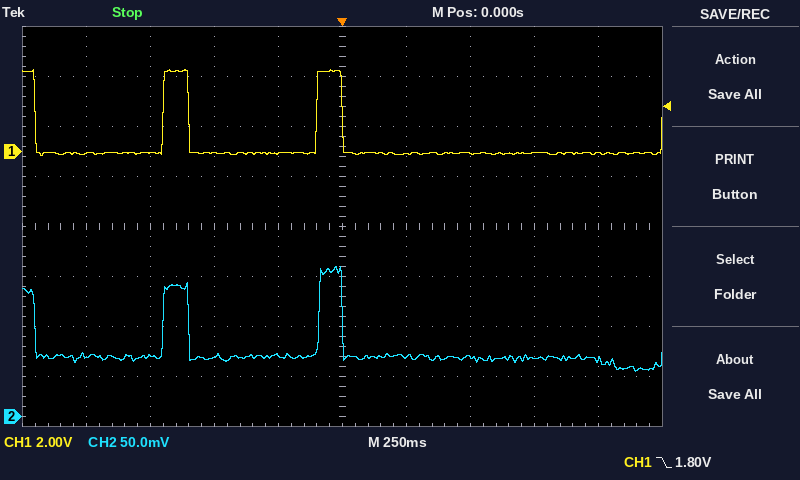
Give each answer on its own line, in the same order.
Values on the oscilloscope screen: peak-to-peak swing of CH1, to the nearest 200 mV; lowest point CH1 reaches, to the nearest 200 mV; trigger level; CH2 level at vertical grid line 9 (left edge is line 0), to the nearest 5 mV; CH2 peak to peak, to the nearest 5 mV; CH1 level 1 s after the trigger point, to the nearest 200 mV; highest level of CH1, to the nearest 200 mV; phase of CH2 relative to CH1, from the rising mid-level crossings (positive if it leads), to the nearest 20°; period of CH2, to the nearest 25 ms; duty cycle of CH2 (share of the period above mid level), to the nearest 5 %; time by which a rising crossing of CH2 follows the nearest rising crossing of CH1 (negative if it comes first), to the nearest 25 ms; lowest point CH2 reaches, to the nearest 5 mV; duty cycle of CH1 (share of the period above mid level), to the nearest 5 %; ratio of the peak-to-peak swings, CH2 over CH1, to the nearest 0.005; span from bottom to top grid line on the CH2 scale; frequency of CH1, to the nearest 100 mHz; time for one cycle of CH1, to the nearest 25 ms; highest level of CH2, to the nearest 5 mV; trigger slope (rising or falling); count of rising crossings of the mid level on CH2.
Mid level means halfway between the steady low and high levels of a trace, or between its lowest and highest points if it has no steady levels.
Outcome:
3.4 V
-200 mV
1.80 V
55 mV
105 mV
0.0 V
3.2 V
0°
600 ms
15 %
0 ms
45 mV
15 %
0.030
400 mV
1.7 Hz
600 ms
150 mV
falling
2
